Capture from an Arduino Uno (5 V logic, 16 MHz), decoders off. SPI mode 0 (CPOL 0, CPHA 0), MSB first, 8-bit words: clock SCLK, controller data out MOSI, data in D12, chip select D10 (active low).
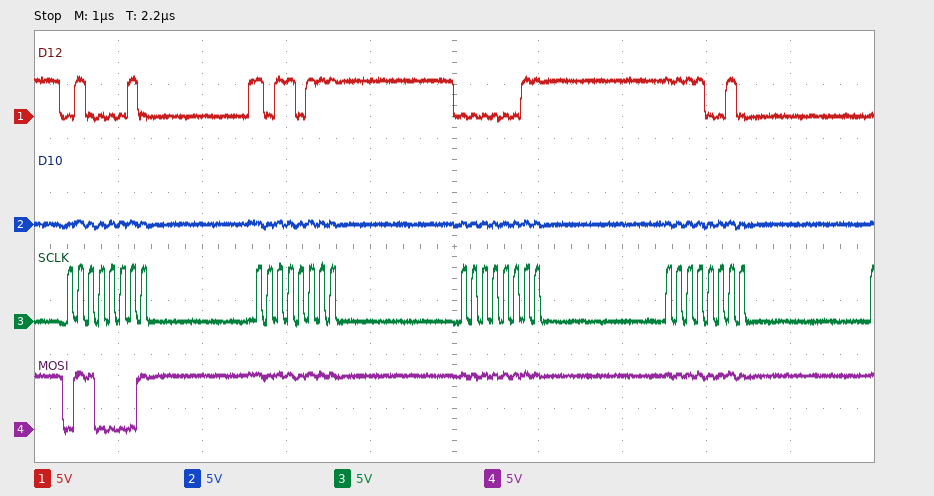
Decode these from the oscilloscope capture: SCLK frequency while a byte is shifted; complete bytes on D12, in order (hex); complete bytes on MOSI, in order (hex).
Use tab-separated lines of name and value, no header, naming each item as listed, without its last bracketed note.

SCLK frequency while a byte is shifted	8 MHz
complete bytes on D12, in order	0x42 0xB7 0x03 0xF2
complete bytes on MOSI, in order	0x61 0xFF 0xFF 0xFF
